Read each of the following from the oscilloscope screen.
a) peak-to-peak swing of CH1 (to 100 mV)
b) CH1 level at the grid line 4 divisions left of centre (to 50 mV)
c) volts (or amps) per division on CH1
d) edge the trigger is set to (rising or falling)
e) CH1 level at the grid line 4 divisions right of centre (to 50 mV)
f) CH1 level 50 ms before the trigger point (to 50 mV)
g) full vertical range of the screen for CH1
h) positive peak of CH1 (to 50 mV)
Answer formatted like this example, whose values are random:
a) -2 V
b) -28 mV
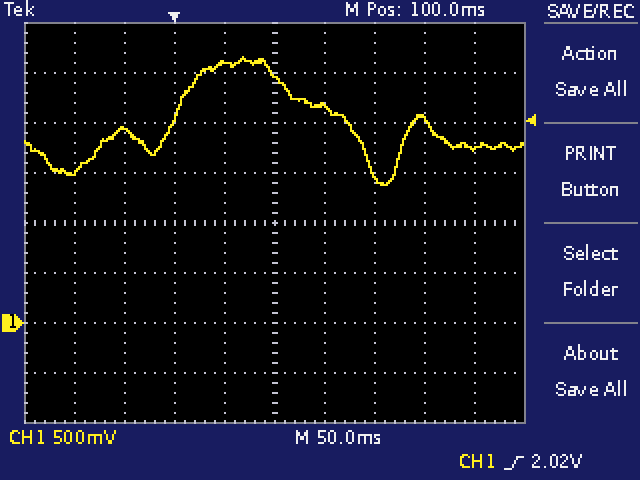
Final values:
a) 1.30 V
b) 1.50 V
c) 500 mV
d) rising
e) 1.75 V
f) 1.95 V
g) 4 V
h) 2.65 V
